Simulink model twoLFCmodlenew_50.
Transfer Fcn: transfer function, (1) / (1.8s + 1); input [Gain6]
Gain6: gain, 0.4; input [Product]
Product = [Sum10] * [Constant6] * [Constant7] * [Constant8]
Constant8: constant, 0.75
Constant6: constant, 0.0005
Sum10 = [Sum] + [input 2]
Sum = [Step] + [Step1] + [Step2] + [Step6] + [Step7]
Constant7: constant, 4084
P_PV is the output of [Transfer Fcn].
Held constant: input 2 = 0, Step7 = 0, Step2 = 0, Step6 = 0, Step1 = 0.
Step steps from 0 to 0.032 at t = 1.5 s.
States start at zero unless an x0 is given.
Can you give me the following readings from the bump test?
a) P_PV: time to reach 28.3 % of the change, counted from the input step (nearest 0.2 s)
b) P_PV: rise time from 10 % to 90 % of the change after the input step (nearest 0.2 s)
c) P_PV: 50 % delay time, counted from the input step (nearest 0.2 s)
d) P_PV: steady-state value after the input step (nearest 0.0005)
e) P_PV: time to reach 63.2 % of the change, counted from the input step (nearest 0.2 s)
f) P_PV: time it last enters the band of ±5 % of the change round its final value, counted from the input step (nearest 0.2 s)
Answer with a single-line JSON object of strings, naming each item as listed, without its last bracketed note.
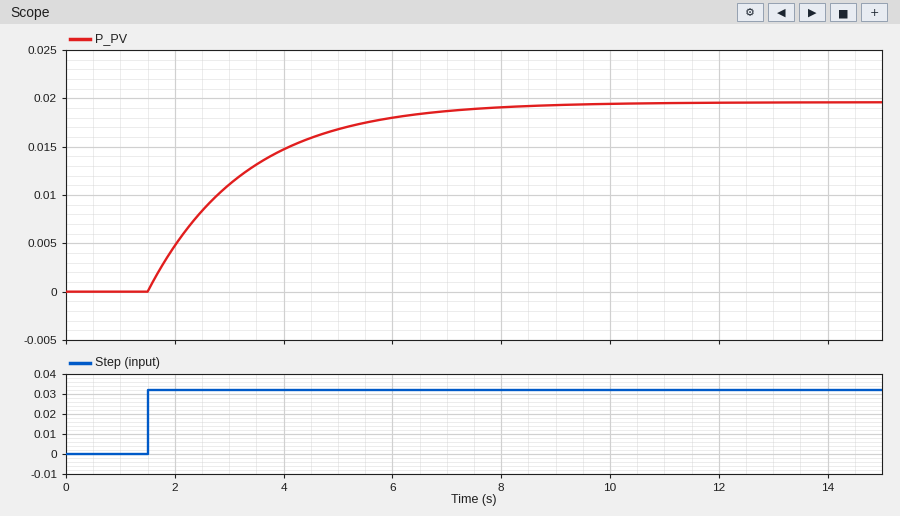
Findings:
{"P_PV: time to reach 28.3 % of the change, counted from the input step": "0.6 s", "P_PV: rise time from 10 % to 90 % of the change after the input step": "4.0 s", "P_PV: 50 % delay time, counted from the input step": "1.2 s", "P_PV: steady-state value after the input step": "0.0195", "P_PV: time to reach 63.2 % of the change, counted from the input step": "1.8 s", "P_PV: time it last enters the band of ±5 % of the change round its final value, counted from the input step": "5.4 s"}
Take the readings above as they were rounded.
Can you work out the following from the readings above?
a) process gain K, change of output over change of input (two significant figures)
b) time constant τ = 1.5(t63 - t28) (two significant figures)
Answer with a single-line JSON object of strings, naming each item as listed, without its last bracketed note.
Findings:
{"process gain K, change of output over change of input": "0.61", "time constant τ = 1.5(t63 - t28)": "1.8 s"}
